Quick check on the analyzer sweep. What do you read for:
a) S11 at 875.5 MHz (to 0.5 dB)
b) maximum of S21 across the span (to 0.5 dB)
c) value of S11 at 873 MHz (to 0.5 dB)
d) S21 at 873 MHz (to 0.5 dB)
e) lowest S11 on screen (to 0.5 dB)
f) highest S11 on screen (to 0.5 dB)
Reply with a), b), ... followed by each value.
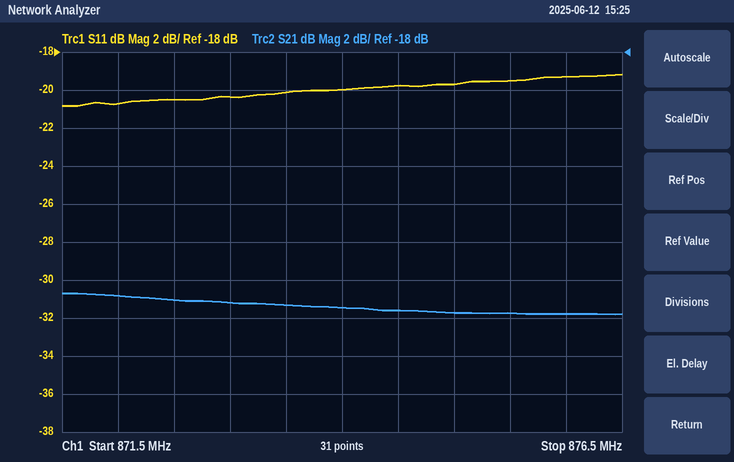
a) -19.5 dB
b) -30.5 dB
c) -20.5 dB
d) -31.0 dB
e) -21.0 dB
f) -19.0 dB
